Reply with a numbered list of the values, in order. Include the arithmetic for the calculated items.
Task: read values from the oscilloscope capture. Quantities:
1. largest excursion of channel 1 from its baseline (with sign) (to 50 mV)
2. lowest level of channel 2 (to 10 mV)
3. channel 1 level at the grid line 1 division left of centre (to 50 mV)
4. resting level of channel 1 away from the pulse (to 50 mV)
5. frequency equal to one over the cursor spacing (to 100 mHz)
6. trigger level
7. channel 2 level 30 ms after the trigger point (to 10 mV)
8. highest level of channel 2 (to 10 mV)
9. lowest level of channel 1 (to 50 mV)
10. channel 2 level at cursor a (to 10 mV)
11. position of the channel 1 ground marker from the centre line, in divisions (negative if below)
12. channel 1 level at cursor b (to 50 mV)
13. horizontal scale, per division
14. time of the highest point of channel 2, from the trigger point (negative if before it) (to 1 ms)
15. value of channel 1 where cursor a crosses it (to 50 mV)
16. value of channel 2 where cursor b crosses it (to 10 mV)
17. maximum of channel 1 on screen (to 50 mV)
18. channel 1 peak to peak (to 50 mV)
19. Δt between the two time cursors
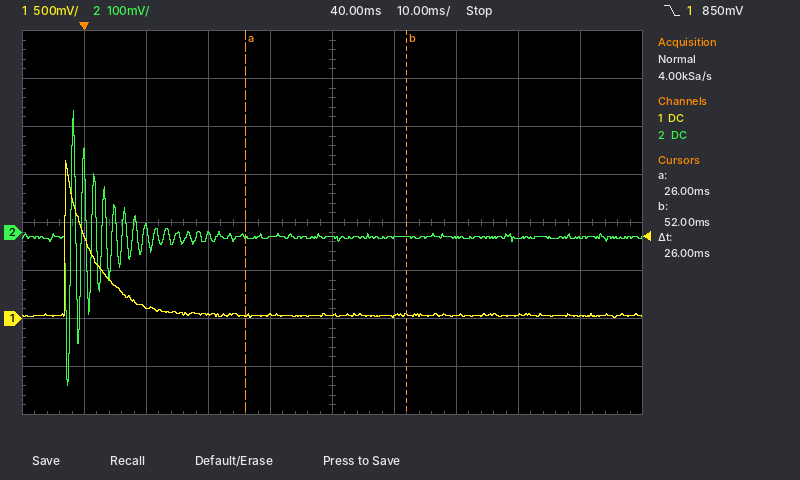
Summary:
1. 1.65 V − (50 mV) = +1.60 V
2. -320 mV
3. 50 mV
4. 50 mV
5. 1 / 26 ms ≈ 38.5 Hz
6. 850 mV
7. -10 mV
8. 250 mV
9. 0 mV
10. -10 mV
11. -2.0 div
12. 50 mV
13. 10 ms
14. -2 ms
15. 50 mV
16. -10 mV
17. 1.65 V
18. 1.65 V − (0 mV) = 1.65 V
19. 26 ms
